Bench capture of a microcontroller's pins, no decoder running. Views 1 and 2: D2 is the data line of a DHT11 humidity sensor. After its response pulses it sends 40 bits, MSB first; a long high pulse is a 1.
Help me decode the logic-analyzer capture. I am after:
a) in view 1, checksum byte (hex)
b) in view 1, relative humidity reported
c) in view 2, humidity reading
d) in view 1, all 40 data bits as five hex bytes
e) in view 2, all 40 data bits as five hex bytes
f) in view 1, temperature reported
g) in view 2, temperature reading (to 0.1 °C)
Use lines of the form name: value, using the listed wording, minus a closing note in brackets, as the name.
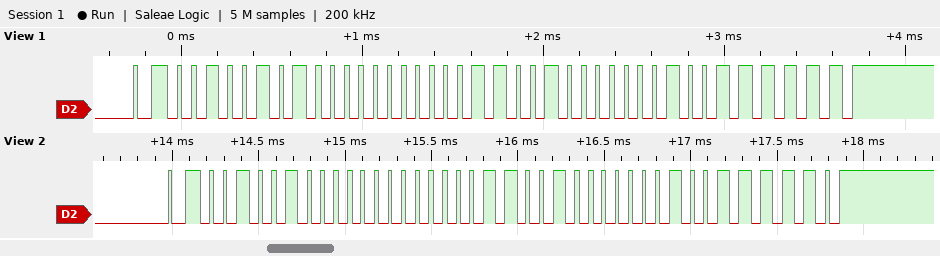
in view 1, checksum byte: 0x3F
in view 1, relative humidity reported: 37 %
in view 2, humidity reading: 36 %
in view 1, all 40 data bits as five hex bytes: 25 00 19 01 3F
in view 2, all 40 data bits as five hex bytes: 24 00 19 01 3E
in view 1, temperature reported: 25.1 °C
in view 2, temperature reading: 25.1 °C
